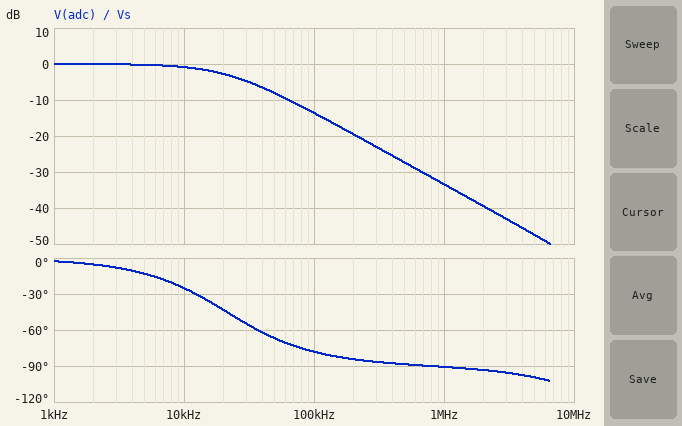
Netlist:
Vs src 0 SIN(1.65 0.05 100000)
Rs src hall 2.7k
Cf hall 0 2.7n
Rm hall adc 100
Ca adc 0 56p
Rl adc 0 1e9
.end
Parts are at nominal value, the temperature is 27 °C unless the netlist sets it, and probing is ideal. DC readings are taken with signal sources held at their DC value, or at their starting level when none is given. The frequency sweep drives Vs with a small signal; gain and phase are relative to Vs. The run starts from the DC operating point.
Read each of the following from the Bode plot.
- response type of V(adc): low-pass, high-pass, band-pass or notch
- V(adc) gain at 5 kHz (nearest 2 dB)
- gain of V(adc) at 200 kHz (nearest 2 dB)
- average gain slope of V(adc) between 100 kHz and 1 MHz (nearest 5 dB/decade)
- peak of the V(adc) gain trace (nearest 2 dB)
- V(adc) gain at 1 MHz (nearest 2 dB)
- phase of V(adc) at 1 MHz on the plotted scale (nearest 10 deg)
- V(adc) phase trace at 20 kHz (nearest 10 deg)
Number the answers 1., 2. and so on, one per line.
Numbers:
1. low-pass
2. 0 dB
3. -20 dB
4. -20 dB/decade
5. 0 dB
6. -34 dB
7. -90 deg
8. -40 deg
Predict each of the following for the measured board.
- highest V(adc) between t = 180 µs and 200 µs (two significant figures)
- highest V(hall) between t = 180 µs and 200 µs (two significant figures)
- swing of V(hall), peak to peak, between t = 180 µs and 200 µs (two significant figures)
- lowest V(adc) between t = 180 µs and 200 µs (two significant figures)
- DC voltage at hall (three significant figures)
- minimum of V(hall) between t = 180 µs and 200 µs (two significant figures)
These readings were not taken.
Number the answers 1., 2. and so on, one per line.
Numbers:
1. 1.7 V
2. 1.7 V
3. 21 mV
4. 1.6 V
5. 1.65 V
6. 1.6 V
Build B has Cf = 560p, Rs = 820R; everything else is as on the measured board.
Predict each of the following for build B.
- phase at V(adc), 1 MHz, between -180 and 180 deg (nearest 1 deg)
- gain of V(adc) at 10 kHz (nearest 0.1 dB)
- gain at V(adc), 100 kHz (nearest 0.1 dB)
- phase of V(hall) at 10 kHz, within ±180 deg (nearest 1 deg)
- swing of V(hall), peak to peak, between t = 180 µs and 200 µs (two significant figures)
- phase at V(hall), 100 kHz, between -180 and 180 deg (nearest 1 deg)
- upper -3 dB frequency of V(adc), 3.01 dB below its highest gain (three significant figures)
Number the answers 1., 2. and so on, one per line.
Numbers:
1. -74 deg
2. 0 dB
3. -0.4 dB
4. -2 deg
5. 95 mV
6. -18 deg
7. 315 kHz
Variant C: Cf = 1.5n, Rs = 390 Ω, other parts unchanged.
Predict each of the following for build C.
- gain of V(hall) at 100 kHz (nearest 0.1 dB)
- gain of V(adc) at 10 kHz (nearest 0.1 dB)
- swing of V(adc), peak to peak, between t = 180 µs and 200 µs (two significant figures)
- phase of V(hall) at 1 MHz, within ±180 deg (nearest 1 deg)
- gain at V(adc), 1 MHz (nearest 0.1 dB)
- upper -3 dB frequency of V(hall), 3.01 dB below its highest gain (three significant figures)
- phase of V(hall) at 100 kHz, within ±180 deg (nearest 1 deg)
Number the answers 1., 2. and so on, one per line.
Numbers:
1. -0.6 dB
2. 0 dB
3. 93 mV
4. -75 deg
5. -11.9 dB
6. 262 kHz
7. -21 deg
